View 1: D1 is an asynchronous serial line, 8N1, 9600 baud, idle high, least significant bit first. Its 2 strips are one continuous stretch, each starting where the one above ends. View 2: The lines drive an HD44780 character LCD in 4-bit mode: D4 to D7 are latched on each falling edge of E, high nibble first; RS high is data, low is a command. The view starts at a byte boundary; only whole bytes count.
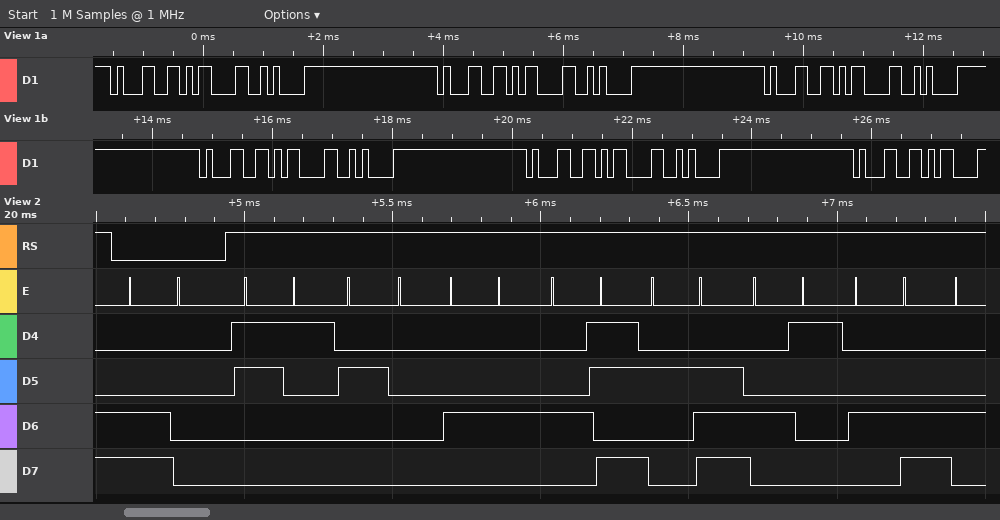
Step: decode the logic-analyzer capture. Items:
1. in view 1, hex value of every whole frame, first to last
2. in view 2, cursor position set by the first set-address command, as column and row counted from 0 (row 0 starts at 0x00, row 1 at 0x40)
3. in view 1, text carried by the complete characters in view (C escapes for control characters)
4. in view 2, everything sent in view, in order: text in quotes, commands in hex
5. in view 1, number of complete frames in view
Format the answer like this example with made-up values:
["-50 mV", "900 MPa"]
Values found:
["31 0D 0A 31 0D 0A 31 0D 0A 31 0D 0A 31 0D 0A 31 0D", "column 0, row 1", "\"1\\r\\n1\\r\\n1\\r\\n1\\r\\n1\\r\\n1\\r\"", "0xC0 \"1 DK.AL\"", "17"]
